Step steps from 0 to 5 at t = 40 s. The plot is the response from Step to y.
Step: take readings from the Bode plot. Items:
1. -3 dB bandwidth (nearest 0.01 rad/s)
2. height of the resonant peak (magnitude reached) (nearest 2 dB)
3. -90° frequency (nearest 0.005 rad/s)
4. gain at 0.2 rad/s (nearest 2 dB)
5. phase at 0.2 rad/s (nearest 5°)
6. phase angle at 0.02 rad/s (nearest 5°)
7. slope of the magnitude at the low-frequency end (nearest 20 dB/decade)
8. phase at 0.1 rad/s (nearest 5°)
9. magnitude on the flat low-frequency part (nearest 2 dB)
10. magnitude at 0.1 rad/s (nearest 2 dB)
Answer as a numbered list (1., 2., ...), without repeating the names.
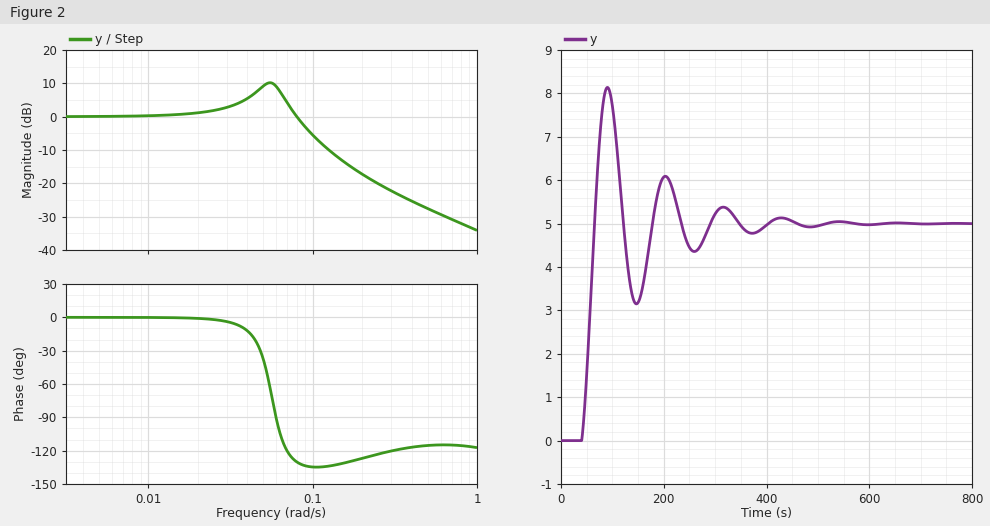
1. 0.09 rad/s
2. 10 dB
3. 0.060 rad/s
4. -18 dB
5. -125°
6. 0°
7. 0 dB/decade
8. -135°
9. 0 dB
10. -6 dB
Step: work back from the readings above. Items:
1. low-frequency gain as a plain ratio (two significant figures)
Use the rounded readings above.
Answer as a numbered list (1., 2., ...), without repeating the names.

1. 1.0
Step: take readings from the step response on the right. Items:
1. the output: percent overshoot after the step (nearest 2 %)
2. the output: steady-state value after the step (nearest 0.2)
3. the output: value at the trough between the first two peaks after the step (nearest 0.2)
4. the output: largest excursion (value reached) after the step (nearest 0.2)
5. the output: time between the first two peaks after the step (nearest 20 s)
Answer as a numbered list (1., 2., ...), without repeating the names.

1. 62 %
2. 5.0
3. 3.2
4. 8.2
5. 120 s
